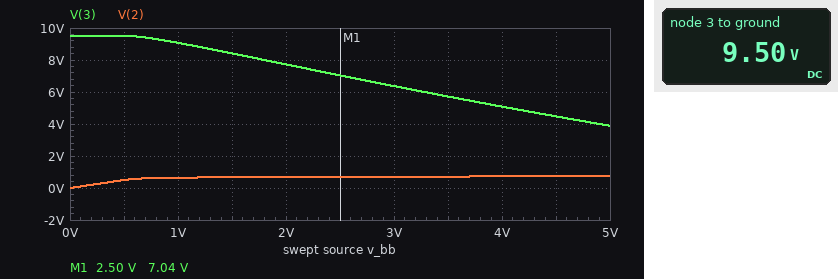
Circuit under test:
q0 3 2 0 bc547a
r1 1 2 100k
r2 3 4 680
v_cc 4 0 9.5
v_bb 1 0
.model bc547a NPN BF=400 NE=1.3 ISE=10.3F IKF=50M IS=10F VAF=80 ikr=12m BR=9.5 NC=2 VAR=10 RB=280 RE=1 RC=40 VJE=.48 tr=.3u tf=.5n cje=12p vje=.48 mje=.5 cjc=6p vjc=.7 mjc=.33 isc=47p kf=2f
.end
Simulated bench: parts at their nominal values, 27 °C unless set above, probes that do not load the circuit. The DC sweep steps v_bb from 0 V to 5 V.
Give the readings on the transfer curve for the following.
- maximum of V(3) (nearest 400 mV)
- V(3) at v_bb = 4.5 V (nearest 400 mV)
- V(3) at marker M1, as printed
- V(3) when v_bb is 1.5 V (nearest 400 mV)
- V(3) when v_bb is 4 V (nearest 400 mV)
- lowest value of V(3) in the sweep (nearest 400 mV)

9.6 V
4.4 V
7.04 V
8.4 V
5.2 V
4.0 V
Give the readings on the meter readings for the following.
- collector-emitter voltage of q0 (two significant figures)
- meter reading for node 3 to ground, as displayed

9.5 V
9.50 V
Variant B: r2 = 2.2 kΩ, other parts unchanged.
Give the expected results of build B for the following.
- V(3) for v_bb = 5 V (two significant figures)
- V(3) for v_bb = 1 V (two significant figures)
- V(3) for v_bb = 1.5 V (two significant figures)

270 mV
8.1 V
6.1 V
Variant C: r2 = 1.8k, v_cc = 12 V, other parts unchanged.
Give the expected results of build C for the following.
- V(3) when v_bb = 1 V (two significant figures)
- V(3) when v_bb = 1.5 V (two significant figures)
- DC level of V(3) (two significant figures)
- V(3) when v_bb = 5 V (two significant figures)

11 V
9.1 V
12 V
400 mV
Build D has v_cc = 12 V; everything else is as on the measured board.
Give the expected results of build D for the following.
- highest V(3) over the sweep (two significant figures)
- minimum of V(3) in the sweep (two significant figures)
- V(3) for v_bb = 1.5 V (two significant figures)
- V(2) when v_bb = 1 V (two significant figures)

12 V
6.2 V
11 V
640 mV
